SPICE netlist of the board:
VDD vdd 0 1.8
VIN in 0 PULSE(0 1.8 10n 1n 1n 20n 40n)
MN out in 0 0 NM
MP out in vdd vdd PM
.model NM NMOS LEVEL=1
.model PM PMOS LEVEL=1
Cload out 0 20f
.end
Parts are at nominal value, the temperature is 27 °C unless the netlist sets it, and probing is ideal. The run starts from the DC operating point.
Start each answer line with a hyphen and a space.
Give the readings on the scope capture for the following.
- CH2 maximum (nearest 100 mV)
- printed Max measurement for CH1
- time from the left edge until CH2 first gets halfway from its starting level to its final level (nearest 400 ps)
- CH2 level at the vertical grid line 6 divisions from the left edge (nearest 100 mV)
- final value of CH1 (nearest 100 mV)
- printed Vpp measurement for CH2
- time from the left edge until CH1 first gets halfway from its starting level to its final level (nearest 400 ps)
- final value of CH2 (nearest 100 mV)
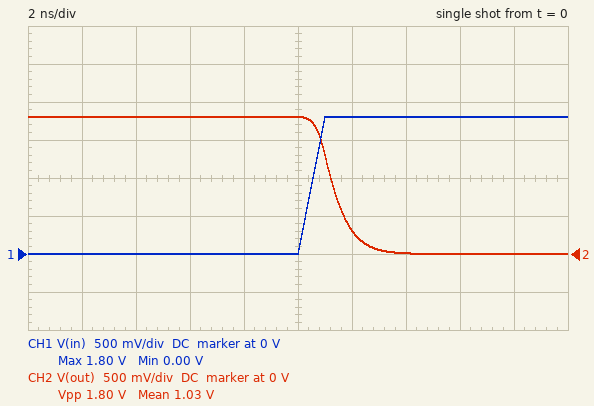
- 1.8 V
- 1.80 V
- 11.2 ns
- 300 mV
- 1.8 V
- 1.80 V
- 10.4 ns
- 0 V
